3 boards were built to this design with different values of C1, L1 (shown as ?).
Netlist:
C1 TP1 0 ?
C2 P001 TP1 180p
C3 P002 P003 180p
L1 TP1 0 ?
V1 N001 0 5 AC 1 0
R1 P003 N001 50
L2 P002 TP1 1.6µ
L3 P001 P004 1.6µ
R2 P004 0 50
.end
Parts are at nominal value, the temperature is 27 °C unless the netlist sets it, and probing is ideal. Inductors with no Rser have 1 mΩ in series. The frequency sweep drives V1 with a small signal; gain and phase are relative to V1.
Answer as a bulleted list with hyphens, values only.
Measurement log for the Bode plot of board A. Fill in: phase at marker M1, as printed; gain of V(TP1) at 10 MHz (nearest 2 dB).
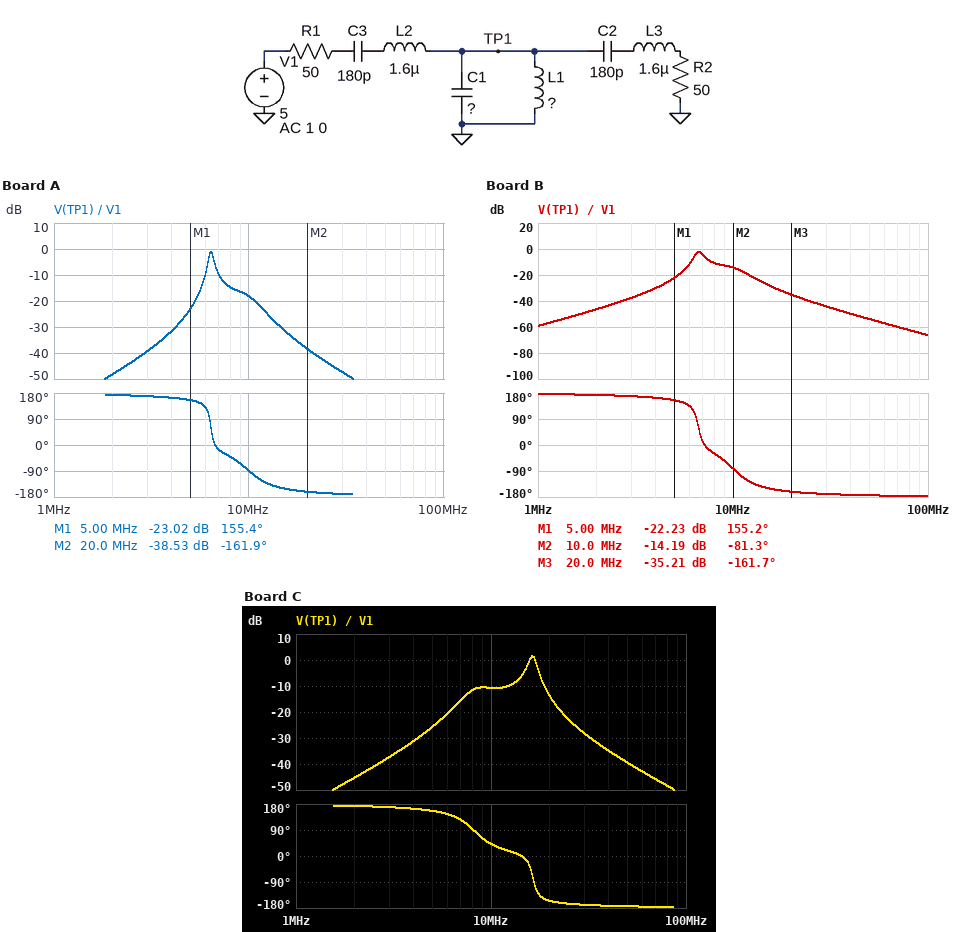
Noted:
- 155.4 deg
- -18 dB
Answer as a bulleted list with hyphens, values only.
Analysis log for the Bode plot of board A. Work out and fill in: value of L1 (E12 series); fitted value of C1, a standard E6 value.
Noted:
- 120 nH
- 4.7 nF
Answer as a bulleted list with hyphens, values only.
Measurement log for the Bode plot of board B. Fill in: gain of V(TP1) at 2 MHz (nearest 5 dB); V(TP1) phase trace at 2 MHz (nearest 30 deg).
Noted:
- -45 dB
- 180 deg
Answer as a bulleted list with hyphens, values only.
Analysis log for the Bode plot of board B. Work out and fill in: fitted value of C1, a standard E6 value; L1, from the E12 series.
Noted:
- 3.3 nF
- 150 nH
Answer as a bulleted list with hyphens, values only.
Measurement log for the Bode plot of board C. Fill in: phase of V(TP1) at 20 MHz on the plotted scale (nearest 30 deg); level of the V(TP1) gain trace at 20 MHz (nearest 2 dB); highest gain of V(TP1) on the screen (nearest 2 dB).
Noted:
- -150 deg
- -14 dB
- 2 dB
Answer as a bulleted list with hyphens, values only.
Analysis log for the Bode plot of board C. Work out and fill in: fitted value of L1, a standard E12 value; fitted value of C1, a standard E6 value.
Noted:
- 180 nH
- 680 pF
